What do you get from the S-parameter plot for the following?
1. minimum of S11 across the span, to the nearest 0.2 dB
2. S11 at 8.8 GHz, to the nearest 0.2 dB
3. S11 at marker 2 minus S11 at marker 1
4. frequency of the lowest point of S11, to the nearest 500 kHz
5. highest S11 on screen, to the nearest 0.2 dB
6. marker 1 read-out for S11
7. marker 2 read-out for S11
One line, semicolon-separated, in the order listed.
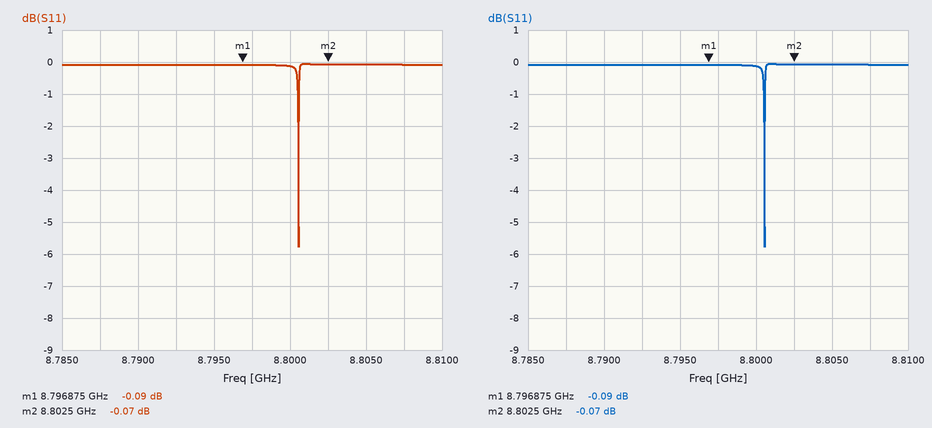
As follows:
-5.8 dB; -0.2 dB; 0.02 dB; 8.8005 GHz; 0.0 dB; -0.09 dB; -0.07 dB
